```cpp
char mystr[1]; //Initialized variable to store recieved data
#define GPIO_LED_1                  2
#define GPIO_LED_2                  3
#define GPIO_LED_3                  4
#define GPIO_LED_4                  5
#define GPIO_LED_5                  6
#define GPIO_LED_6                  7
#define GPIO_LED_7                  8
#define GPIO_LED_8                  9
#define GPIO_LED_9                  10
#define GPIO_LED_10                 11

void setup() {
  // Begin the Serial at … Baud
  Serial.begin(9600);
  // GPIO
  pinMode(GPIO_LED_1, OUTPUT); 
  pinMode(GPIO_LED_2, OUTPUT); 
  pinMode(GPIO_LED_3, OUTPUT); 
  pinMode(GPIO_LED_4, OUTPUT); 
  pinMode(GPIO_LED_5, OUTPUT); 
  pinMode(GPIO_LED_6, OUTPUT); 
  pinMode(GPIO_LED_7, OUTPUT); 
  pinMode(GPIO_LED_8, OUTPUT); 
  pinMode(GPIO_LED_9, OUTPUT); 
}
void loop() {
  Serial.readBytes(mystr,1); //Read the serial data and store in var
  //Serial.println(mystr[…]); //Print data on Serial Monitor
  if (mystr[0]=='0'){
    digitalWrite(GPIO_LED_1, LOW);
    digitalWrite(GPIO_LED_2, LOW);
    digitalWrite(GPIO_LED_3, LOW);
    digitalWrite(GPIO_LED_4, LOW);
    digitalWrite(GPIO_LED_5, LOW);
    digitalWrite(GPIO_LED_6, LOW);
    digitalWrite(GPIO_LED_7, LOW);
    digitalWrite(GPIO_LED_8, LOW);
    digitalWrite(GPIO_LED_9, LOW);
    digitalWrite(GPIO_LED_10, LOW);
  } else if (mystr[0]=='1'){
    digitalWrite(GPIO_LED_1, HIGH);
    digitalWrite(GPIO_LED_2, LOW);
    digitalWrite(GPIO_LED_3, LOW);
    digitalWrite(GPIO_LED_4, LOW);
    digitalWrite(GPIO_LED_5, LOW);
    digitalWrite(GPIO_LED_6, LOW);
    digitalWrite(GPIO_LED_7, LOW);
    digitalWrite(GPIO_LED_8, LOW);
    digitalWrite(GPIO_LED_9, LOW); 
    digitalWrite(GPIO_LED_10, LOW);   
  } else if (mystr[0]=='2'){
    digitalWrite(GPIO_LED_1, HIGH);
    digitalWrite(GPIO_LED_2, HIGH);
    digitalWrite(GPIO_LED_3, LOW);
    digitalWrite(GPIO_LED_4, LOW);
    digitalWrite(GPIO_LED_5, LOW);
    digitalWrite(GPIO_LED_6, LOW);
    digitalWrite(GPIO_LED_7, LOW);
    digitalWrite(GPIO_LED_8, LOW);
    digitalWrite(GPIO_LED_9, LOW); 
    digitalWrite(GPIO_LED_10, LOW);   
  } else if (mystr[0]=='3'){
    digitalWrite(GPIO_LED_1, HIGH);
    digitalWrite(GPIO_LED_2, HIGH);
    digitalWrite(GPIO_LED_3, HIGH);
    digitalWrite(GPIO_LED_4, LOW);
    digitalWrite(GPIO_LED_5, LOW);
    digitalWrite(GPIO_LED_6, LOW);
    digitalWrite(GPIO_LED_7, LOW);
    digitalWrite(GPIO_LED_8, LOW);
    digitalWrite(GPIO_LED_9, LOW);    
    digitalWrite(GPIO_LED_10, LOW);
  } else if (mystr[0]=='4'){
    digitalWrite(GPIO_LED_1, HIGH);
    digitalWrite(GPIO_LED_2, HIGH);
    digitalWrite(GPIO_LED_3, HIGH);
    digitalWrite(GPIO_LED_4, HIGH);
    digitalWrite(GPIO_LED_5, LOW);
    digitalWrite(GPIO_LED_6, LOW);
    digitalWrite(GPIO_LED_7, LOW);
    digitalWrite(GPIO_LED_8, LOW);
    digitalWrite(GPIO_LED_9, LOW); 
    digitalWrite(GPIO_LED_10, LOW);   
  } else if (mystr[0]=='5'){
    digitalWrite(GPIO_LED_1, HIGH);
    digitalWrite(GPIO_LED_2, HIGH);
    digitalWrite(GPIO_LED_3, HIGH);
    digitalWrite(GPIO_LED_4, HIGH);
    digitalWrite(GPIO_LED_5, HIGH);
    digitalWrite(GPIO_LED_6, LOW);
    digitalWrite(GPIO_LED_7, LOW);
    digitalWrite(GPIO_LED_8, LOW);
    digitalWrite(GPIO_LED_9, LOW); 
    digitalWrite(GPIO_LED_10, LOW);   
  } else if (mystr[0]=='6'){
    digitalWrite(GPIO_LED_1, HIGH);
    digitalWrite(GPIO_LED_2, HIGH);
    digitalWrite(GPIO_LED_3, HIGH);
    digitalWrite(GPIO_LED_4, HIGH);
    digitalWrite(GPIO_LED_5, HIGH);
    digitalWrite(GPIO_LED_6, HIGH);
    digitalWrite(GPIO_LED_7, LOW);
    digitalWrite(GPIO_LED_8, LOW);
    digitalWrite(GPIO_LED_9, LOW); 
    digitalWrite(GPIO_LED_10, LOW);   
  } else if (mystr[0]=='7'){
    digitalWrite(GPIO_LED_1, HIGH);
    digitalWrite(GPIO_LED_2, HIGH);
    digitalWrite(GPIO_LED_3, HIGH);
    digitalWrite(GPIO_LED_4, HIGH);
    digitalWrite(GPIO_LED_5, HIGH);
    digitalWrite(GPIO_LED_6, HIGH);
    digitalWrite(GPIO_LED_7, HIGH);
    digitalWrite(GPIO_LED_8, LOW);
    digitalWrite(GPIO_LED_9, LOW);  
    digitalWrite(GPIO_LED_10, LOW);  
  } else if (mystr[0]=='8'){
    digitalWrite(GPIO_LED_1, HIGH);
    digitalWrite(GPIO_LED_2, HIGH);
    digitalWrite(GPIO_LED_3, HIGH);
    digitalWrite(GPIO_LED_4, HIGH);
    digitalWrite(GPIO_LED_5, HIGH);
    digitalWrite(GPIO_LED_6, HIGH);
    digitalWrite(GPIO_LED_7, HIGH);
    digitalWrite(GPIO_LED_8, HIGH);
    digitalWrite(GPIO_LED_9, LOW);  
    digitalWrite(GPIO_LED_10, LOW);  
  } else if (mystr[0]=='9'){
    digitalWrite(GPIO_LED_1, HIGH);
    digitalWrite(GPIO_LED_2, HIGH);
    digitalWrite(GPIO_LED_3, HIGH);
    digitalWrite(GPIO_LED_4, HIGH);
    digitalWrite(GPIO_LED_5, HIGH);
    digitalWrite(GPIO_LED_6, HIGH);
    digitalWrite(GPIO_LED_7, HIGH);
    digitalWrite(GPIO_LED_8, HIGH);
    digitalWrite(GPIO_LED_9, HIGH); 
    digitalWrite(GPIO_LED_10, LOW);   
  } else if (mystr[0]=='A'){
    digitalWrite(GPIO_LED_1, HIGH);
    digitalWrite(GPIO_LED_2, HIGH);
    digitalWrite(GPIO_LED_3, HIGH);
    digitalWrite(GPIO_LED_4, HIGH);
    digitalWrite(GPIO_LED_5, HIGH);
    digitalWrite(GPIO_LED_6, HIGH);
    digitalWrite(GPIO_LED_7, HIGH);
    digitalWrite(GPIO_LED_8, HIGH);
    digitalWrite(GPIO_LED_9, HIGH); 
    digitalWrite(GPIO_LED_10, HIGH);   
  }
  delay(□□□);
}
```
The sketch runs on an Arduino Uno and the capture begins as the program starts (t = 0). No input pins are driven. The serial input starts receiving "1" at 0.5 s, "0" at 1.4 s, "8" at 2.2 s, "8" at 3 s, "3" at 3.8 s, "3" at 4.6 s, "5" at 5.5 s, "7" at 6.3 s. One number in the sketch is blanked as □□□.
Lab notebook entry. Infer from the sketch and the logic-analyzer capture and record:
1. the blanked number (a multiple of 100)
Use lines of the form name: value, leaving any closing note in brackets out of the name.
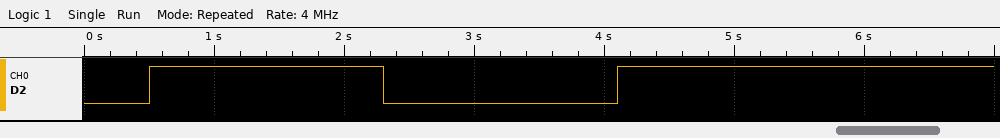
the blanked number: 1800
